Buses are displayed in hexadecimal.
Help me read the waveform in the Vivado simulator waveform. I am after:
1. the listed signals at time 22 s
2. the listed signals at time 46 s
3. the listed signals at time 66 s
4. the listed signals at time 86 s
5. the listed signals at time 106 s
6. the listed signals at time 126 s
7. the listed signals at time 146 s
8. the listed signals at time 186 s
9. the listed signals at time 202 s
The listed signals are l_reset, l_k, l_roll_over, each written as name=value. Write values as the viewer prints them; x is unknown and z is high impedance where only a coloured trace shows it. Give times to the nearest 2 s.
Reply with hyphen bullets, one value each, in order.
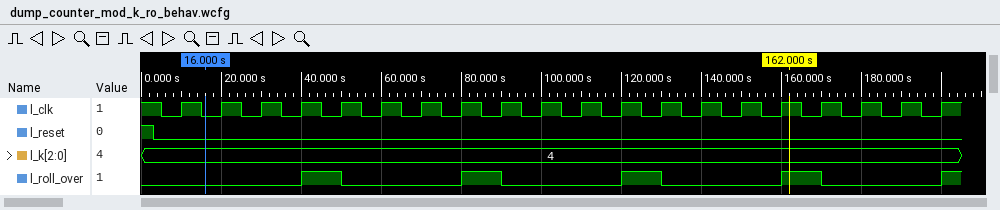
- l_reset=0, l_k=4, l_roll_over=0
- l_reset=0, l_k=4, l_roll_over=1
- l_reset=0, l_k=4, l_roll_over=0
- l_reset=0, l_k=4, l_roll_over=1
- l_reset=0, l_k=4, l_roll_over=0
- l_reset=0, l_k=4, l_roll_over=1
- l_reset=0, l_k=4, l_roll_over=0
- l_reset=0, l_k=4, l_roll_over=0
- l_reset=0, l_k=4, l_roll_over=1
